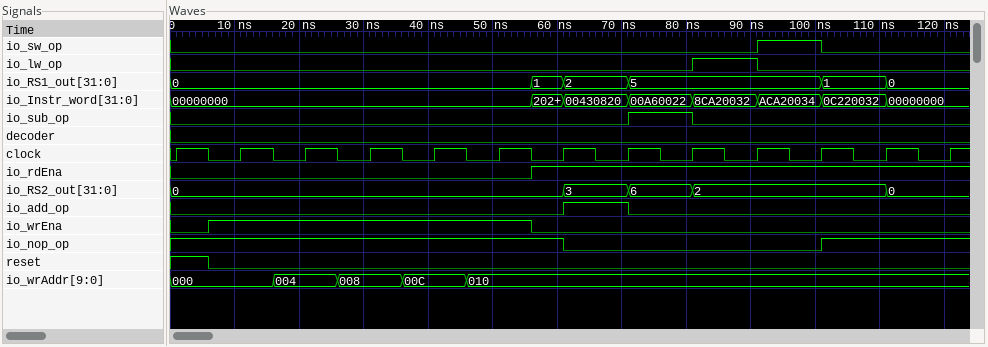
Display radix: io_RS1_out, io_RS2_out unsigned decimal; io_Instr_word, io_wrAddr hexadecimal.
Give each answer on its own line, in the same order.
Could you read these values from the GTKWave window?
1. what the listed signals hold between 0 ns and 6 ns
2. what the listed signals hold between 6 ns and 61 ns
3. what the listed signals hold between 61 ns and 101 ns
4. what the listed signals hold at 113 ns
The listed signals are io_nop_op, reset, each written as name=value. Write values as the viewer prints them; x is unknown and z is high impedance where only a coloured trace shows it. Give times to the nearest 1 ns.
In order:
io_nop_op=1, reset=1
io_nop_op=1, reset=0
io_nop_op=0, reset=0
io_nop_op=1, reset=0
